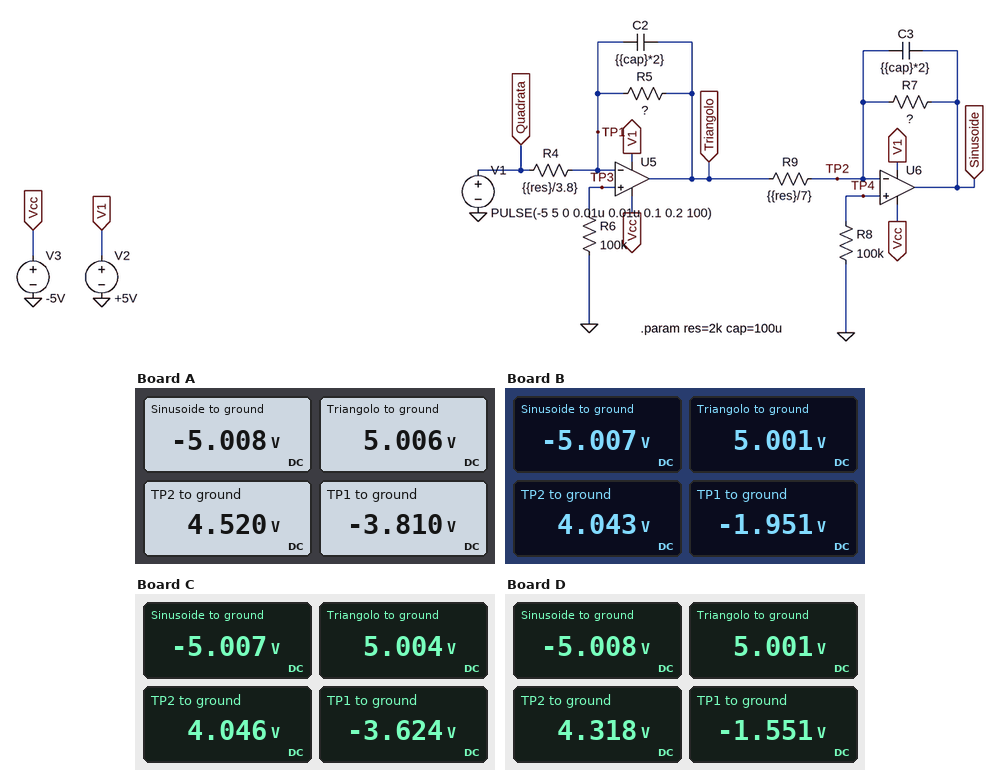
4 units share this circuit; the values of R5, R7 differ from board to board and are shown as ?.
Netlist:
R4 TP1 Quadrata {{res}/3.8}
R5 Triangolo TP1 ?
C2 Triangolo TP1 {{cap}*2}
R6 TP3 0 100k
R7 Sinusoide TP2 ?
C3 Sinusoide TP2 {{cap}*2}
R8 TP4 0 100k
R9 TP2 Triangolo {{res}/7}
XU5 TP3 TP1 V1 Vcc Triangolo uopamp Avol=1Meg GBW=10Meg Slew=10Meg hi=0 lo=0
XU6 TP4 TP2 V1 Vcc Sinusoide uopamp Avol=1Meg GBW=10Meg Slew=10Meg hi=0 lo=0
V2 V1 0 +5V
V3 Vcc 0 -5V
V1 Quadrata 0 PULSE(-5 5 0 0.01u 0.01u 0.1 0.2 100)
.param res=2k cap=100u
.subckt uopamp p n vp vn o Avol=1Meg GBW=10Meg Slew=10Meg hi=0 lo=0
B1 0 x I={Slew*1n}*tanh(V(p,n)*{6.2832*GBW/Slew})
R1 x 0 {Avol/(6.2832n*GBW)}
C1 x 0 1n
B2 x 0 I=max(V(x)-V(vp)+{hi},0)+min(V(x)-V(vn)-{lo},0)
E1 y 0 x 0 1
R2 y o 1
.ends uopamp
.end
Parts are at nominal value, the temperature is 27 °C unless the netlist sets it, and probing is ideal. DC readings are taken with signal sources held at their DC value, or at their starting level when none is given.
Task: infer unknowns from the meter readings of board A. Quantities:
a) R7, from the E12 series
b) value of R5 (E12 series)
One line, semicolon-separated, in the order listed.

5.6 kΩ; 3.9 kΩ
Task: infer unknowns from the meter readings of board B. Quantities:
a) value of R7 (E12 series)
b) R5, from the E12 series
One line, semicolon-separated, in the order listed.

2.7 kΩ; 1.2 kΩ
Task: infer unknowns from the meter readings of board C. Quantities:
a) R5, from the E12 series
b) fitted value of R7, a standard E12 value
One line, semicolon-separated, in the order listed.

3.3 kΩ; 2.7 kΩ
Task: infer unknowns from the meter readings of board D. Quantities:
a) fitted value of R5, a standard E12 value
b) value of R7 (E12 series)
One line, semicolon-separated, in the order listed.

1 kΩ; 3.9 kΩ
